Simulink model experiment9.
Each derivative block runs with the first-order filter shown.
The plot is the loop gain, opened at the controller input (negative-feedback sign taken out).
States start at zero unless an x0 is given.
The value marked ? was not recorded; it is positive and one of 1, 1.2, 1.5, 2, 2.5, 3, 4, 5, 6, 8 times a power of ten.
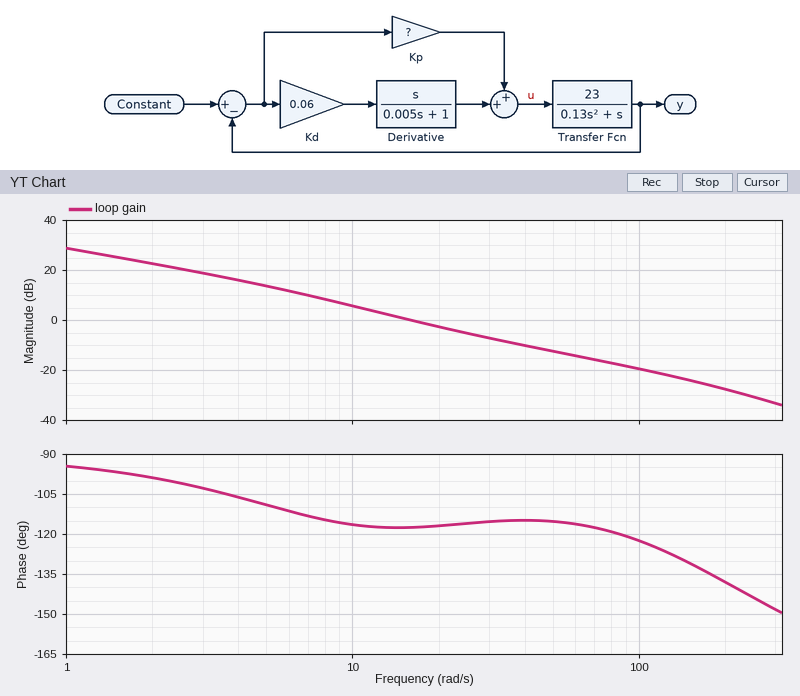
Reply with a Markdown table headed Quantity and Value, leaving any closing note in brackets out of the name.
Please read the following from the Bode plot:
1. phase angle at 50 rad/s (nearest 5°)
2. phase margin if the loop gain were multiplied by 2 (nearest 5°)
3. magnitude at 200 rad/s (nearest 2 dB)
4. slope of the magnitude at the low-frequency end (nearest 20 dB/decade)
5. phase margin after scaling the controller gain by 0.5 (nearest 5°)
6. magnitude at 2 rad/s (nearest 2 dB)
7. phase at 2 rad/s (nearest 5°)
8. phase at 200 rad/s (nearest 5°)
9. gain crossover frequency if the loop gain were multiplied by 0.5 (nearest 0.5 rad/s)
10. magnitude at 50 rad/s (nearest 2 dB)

| Quantity | Value |
|---|---|
| phase angle at 50 rad/s | -115° |
| phase margin if the loop gain were multiplied by 2 | 65° |
| magnitude at 200 rad/s | -28 dB |
| slope of the magnitude at the low-frequency end | -20 dB/decade |
| phase margin after scaling the controller gain by 0.5 | 65° |
| magnitude at 2 rad/s | 22 dB |
| phase at 2 rad/s | -100° |
| phase at 200 rad/s | -140° |
| gain crossover frequency if the loop gain were multiplied by 0.5 | 9.5 rad/s |
| magnitude at 50 rad/s | -12 dB |
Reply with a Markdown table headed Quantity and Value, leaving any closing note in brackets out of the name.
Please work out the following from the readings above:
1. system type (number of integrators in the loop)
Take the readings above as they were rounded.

| Quantity | Value |
|---|---|
| system type | 1 |
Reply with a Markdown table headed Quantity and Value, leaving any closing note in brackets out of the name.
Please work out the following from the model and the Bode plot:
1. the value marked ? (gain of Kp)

| Quantity | Value |
|---|---|
| the value marked ? | 1.2 |
